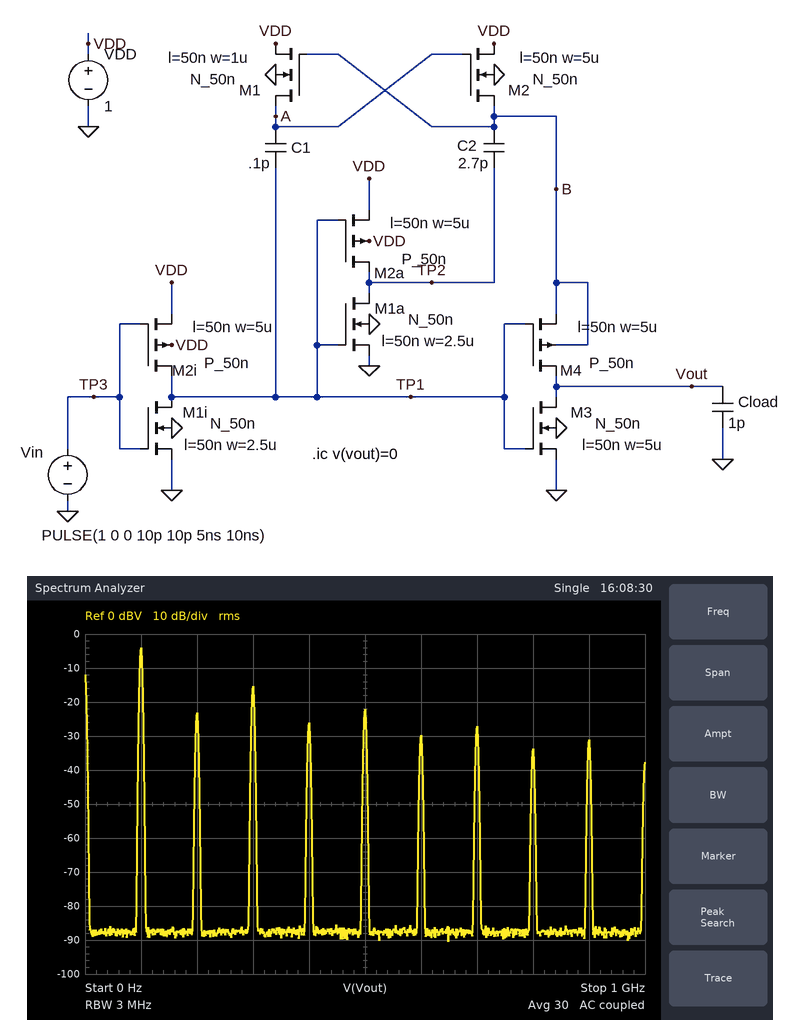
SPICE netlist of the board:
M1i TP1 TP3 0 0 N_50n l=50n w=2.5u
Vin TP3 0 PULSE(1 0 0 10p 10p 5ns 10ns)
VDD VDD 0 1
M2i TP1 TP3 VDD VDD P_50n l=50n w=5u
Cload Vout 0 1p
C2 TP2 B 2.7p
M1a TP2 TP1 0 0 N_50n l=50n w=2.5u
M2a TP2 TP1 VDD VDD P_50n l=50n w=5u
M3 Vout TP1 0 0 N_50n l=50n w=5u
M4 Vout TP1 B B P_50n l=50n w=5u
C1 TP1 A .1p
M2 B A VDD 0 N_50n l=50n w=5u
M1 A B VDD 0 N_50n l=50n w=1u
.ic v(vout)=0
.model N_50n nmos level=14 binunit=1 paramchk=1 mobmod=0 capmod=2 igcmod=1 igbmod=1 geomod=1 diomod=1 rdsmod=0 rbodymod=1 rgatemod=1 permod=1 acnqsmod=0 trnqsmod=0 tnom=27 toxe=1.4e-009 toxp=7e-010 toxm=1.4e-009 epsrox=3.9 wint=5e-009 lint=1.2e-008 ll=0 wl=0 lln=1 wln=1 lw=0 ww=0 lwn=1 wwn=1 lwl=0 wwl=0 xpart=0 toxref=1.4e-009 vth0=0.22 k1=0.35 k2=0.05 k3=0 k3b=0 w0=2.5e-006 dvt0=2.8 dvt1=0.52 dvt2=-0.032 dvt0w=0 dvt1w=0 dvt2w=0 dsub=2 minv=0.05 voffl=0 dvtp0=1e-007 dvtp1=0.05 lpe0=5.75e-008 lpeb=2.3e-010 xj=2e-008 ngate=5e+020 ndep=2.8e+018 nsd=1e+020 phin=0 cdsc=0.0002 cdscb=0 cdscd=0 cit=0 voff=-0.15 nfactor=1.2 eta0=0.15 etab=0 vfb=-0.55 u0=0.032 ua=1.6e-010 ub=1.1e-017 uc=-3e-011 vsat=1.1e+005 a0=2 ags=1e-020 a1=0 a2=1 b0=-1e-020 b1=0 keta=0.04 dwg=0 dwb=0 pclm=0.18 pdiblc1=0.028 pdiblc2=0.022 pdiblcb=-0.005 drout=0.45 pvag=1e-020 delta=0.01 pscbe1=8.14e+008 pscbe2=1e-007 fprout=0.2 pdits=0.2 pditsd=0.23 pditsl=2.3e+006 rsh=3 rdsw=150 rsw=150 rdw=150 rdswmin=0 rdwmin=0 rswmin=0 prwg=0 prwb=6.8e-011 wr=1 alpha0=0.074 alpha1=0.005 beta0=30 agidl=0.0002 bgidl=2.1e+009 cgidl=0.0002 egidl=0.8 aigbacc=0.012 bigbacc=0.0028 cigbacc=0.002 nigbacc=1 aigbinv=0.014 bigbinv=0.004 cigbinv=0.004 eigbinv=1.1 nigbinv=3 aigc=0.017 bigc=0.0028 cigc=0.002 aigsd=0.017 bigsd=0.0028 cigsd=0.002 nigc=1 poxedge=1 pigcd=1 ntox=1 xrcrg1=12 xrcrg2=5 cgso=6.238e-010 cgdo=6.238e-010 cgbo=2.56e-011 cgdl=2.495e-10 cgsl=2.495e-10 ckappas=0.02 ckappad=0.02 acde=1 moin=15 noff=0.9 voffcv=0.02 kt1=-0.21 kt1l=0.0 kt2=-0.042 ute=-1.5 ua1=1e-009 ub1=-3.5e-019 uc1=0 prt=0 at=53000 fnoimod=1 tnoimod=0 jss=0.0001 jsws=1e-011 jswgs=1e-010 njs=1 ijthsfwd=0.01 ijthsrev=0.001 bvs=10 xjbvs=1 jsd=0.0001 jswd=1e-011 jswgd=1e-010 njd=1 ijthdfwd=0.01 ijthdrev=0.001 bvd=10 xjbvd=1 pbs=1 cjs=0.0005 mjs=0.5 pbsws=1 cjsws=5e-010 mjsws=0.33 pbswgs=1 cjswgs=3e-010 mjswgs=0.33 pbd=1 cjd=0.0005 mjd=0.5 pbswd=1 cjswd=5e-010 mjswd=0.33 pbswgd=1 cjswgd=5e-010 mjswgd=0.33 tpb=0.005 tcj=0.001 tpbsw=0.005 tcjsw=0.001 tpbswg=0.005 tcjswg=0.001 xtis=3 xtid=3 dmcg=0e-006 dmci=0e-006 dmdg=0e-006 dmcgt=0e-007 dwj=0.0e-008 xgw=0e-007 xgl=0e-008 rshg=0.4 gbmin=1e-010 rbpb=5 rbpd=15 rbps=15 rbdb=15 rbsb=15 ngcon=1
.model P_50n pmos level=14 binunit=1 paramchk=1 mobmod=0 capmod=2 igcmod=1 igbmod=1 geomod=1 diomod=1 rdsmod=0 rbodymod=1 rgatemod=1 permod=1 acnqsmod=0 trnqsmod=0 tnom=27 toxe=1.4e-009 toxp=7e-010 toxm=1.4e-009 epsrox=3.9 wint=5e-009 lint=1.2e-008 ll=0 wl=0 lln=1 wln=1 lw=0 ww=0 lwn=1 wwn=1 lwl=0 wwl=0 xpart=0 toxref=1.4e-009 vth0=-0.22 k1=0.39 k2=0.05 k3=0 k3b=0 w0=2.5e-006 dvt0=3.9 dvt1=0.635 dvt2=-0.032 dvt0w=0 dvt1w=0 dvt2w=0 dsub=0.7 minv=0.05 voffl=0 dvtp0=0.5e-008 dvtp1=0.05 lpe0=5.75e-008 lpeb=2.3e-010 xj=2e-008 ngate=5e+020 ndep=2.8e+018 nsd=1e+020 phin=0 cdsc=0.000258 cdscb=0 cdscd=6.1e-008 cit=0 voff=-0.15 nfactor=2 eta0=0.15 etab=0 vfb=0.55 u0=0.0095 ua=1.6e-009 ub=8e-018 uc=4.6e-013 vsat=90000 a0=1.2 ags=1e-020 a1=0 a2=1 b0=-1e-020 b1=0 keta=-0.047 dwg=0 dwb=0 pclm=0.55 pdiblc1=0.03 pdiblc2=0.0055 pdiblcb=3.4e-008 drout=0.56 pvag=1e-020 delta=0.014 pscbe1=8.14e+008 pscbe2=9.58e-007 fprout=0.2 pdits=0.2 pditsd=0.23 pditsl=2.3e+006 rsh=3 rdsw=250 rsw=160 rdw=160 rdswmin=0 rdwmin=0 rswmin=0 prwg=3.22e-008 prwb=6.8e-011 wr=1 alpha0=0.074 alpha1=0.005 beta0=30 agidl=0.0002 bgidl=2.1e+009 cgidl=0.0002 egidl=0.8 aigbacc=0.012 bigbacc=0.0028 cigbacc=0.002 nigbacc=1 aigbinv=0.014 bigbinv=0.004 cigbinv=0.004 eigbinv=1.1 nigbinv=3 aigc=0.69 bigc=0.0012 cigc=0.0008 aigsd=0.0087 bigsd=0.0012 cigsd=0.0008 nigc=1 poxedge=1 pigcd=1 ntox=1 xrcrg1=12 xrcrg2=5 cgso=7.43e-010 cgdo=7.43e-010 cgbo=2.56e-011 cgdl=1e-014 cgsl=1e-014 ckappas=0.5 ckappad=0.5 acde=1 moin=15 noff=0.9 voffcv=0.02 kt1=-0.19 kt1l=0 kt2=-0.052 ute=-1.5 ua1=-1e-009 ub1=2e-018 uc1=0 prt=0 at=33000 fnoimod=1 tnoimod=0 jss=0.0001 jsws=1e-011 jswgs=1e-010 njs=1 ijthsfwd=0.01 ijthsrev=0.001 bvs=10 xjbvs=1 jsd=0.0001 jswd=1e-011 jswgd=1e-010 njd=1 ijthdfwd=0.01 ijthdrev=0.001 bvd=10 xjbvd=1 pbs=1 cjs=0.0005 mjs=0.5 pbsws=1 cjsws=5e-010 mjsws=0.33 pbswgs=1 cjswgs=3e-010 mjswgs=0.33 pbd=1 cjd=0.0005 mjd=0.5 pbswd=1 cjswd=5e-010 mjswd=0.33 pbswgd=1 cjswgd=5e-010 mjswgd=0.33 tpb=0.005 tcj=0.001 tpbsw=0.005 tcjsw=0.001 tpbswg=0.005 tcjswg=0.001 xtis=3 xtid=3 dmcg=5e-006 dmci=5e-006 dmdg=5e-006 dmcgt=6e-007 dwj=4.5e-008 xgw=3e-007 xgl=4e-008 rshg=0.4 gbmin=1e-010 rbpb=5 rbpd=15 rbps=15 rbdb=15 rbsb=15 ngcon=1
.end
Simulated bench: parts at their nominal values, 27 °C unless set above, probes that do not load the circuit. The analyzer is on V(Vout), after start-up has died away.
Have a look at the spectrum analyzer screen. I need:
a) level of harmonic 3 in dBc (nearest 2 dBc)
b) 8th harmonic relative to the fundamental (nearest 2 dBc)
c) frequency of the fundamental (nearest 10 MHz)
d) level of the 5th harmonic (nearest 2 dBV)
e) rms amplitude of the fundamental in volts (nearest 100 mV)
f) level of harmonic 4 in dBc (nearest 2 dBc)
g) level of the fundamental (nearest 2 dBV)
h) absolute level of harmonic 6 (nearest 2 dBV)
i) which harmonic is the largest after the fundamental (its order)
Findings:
-12 dBc
-30 dBc
100 MHz
-22 dBV
600 mV
-22 dBc
-4 dBV
-30 dBV
3
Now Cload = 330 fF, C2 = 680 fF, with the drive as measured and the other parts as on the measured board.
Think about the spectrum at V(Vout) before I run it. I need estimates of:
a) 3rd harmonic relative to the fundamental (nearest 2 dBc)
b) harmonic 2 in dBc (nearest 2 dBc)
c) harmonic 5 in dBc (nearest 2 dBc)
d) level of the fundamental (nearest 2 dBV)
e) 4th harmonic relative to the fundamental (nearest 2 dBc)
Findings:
-10 dBc
-28 dBc
-14 dBc
-4 dBV
-28 dBc
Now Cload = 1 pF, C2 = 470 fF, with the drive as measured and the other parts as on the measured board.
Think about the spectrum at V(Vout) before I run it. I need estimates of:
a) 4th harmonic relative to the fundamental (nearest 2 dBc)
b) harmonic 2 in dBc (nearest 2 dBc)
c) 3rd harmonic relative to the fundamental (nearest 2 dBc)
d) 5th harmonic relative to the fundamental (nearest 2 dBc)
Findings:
-26 dBc
-26 dBc
-10 dBc
-16 dBc
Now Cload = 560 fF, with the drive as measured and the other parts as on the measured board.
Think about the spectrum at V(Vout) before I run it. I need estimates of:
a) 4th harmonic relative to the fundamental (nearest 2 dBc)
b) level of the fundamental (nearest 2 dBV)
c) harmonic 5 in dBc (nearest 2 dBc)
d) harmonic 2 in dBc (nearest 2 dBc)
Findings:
-24 dBc
-2 dBV
-16 dBc
-22 dBc
